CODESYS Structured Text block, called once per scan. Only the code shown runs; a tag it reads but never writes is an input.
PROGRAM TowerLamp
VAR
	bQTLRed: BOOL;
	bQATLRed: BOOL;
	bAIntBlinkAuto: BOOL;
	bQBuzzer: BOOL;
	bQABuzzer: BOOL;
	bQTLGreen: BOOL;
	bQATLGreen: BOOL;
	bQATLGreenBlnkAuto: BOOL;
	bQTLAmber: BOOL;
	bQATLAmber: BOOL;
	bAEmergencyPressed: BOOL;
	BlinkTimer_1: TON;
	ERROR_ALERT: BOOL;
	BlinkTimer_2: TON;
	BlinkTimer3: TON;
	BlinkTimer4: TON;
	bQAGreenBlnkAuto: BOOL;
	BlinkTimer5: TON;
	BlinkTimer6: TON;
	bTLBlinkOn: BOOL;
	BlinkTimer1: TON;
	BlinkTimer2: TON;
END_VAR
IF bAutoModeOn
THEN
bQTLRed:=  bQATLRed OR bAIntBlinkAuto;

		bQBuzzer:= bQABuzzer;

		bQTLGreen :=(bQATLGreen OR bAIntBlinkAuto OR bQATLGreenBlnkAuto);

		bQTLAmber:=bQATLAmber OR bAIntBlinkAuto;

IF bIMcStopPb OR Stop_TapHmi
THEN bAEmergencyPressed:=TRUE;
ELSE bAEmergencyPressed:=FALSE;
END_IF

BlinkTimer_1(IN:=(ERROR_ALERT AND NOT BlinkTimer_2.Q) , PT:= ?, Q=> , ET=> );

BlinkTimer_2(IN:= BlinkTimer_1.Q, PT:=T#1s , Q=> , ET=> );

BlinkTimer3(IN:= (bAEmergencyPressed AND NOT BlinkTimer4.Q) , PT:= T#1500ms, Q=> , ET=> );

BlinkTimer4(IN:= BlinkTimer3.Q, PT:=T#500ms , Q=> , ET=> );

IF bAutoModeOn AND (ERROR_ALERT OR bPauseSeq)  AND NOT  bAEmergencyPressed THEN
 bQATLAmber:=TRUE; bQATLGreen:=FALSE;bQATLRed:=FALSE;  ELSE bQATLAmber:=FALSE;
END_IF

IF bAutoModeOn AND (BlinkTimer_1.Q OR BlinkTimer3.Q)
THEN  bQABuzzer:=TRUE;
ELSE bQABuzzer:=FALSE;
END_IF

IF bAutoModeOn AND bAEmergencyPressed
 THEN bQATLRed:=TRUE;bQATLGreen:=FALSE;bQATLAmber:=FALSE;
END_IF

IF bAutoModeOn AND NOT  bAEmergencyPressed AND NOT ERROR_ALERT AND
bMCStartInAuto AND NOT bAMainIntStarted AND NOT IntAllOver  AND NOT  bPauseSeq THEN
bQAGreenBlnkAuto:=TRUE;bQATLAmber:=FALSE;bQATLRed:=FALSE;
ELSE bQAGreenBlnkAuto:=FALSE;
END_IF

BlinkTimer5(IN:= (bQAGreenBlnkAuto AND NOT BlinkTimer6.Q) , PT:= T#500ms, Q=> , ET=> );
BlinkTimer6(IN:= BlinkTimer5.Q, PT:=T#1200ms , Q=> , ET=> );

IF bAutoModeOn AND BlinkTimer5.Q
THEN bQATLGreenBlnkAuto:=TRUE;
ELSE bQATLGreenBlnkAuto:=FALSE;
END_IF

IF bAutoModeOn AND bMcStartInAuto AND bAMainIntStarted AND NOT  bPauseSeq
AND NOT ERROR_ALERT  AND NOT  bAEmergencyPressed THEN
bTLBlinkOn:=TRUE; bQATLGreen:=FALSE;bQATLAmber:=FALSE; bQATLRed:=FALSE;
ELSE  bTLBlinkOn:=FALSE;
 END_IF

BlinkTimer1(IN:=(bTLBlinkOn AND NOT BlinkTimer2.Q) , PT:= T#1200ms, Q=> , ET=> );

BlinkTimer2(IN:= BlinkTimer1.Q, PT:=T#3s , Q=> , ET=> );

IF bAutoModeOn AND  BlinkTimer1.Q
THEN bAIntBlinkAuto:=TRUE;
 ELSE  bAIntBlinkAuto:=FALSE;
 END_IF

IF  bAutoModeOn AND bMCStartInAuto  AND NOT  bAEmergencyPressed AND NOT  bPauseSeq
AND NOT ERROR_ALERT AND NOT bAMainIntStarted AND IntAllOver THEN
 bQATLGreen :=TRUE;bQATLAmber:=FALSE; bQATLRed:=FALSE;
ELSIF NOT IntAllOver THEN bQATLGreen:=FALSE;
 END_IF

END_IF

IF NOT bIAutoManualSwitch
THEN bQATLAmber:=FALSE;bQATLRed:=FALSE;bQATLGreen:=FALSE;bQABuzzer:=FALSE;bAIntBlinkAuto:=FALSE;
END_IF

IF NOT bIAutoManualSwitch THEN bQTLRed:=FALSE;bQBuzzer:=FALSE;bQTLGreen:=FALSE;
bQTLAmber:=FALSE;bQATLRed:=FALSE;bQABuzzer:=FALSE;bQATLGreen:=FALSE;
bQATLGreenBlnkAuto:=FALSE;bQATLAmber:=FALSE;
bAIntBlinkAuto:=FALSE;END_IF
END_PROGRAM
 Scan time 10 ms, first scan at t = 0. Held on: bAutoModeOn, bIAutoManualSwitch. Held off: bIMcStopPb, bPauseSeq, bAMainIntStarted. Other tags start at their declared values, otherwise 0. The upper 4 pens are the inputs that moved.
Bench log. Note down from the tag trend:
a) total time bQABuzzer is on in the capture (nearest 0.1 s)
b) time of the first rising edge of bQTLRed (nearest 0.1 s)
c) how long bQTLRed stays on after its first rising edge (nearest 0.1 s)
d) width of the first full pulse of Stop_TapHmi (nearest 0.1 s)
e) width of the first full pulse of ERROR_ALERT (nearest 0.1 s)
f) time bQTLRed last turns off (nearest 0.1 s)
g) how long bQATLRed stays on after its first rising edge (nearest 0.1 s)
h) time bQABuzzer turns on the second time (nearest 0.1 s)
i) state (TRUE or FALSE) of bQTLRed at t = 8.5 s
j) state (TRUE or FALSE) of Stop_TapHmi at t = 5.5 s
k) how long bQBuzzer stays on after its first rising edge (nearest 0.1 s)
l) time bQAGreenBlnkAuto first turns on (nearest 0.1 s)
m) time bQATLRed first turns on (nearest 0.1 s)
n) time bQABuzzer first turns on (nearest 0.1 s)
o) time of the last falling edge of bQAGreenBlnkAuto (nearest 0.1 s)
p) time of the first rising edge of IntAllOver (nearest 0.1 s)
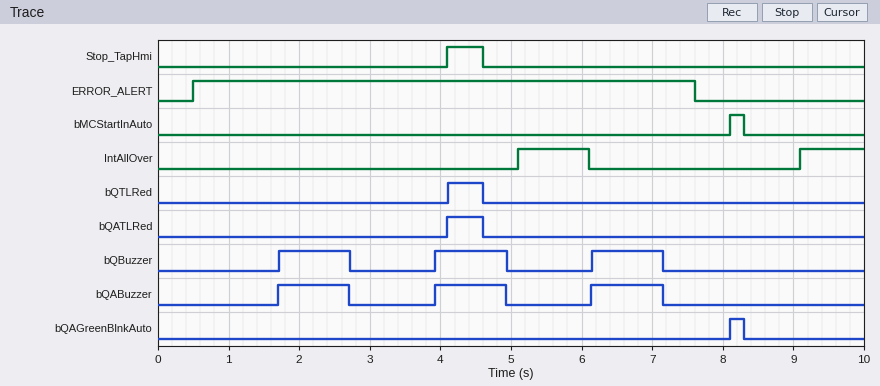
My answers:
3.0 s
4.1 s
0.5 s
0.5 s
7.1 s
4.6 s
0.5 s
3.9 s
FALSE
FALSE
1.0 s
8.1 s
4.1 s
1.7 s
8.3 s
5.1 s
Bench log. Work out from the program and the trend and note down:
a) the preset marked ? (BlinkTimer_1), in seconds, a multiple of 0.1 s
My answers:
1.2 s
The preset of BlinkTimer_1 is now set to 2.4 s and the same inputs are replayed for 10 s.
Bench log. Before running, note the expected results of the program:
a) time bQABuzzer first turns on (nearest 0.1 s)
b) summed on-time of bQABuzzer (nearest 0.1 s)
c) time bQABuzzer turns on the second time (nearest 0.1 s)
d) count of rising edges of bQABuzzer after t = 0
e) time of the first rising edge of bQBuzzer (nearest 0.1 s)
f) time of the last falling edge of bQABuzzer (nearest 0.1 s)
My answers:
2.9 s
2.0 s
6.3 s
2
2.9 s
7.3 s
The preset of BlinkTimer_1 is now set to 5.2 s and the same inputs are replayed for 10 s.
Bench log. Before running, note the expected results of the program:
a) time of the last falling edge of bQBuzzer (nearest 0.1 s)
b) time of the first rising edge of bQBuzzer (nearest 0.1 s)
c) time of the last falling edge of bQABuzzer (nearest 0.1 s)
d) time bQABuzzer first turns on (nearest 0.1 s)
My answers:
6.7 s
5.7 s
6.7 s
5.7 s
